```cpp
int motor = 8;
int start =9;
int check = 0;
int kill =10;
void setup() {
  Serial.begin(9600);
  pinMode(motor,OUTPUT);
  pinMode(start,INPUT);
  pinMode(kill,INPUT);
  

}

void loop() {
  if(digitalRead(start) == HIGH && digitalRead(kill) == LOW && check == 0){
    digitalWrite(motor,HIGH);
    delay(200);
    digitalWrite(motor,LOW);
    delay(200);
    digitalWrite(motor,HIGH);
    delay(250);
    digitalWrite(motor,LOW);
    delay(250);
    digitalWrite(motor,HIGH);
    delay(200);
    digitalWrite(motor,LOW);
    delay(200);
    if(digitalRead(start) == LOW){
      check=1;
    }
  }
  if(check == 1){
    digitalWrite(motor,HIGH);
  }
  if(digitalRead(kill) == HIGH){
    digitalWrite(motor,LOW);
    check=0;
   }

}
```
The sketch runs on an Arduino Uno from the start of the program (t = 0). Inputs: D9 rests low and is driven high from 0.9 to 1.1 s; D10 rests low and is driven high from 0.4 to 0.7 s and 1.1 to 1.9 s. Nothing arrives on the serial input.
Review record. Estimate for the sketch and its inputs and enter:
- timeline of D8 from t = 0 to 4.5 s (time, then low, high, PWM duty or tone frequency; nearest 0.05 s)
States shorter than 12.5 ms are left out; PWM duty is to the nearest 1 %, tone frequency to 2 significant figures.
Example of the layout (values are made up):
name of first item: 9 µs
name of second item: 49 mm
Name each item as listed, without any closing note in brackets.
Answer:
timeline of D8 from t = 0 to 4.5 s: 0 s low; 0.9 s high; 1.1 s low; 1.3 s high; 1.55 s low; 1.8 s high; 2 s low; 2.2 s high
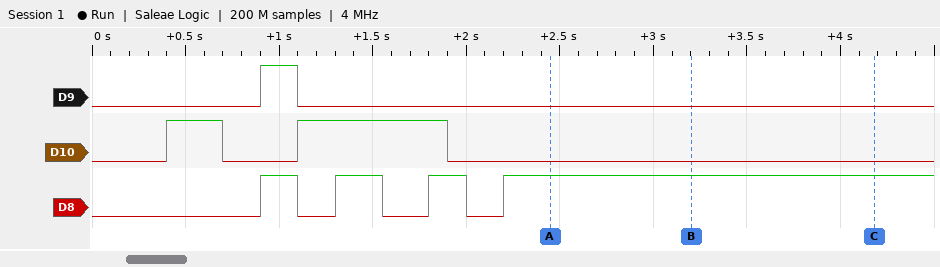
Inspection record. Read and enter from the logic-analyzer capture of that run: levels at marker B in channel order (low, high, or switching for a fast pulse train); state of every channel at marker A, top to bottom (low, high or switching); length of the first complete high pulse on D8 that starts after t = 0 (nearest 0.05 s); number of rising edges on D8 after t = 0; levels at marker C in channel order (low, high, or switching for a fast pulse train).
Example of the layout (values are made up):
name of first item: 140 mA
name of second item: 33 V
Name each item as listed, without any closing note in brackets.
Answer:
levels at marker B in channel order: D9 low, D10 low, D8 high
state of every channel at marker A, top to bottom: D9 low, D10 low, D8 high
length of the first complete high pulse on D8 that starts after t = 0: 0.20 s
number of rising edges on D8 after t = 0: 4
levels at marker C in channel order: D9 low, D10 low, D8 high
